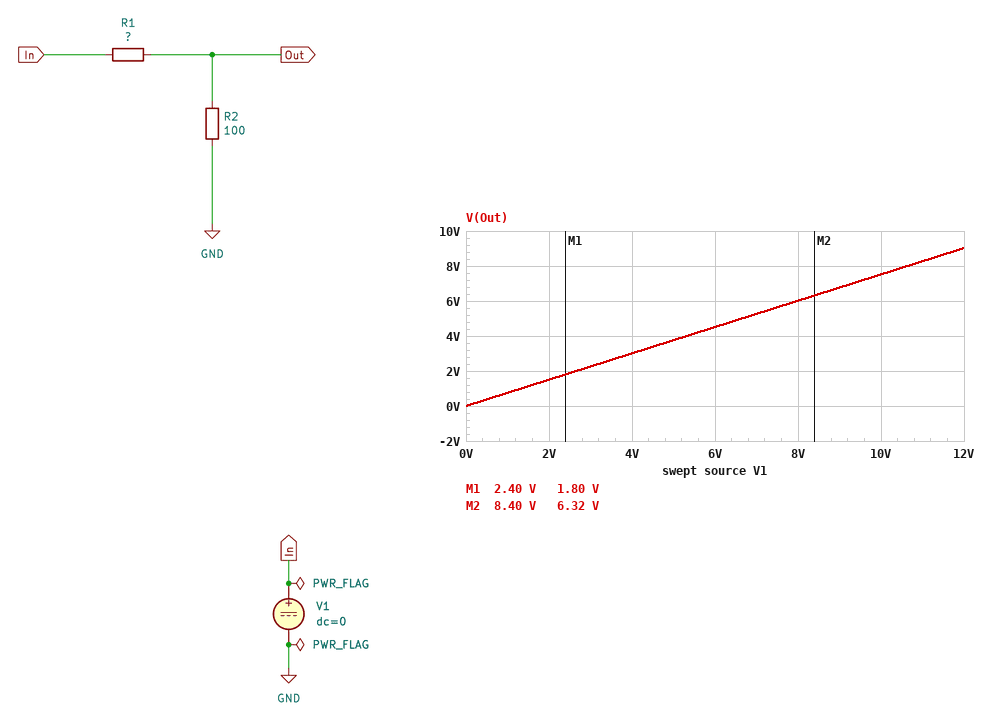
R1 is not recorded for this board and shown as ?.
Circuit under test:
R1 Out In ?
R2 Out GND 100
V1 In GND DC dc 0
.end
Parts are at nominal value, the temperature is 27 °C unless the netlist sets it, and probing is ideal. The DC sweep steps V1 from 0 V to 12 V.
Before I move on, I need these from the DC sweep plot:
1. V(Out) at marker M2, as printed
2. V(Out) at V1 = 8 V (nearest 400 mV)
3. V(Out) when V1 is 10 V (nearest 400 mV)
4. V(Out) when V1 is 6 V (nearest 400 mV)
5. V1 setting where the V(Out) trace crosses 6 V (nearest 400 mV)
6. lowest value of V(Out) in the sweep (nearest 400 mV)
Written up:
6.32 V
6.0 V
7.6 V
4.4 V
8.0 V
0 V
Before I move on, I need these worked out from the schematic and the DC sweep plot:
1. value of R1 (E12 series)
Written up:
33 Ω
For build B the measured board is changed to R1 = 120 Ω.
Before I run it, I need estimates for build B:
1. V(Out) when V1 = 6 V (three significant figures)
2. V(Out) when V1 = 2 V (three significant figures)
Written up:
2.73 V
909 mV
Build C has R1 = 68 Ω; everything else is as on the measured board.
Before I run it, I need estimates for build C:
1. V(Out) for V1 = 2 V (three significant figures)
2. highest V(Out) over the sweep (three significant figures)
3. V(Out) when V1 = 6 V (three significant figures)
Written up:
1.19 V
7.14 V
3.57 V
